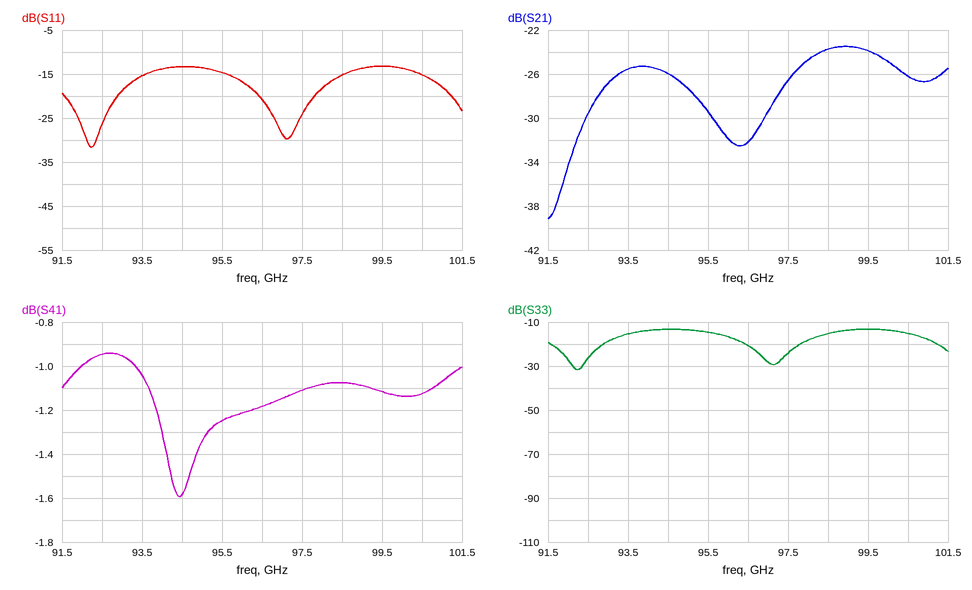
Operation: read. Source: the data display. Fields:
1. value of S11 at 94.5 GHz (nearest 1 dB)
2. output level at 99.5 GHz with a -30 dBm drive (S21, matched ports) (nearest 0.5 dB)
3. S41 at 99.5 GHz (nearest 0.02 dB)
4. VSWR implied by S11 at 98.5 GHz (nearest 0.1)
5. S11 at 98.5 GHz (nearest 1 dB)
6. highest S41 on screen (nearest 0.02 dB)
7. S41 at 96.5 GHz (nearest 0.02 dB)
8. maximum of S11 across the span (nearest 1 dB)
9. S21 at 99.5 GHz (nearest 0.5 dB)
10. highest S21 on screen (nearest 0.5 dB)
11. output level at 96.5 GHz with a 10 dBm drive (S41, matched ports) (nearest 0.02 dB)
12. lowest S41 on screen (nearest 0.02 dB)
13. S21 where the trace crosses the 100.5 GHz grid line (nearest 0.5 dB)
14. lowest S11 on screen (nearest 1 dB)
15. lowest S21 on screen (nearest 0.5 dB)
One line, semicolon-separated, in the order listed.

-13 dB; -54.0 dBm; -1.12 dB; 1.4; -15 dB; -0.94 dB; -1.18 dB; -13 dB; -24.0 dB; -23.5 dB; 8.82 dBm; -1.60 dB; -26.0 dB; -32 dB; -39.0 dB
